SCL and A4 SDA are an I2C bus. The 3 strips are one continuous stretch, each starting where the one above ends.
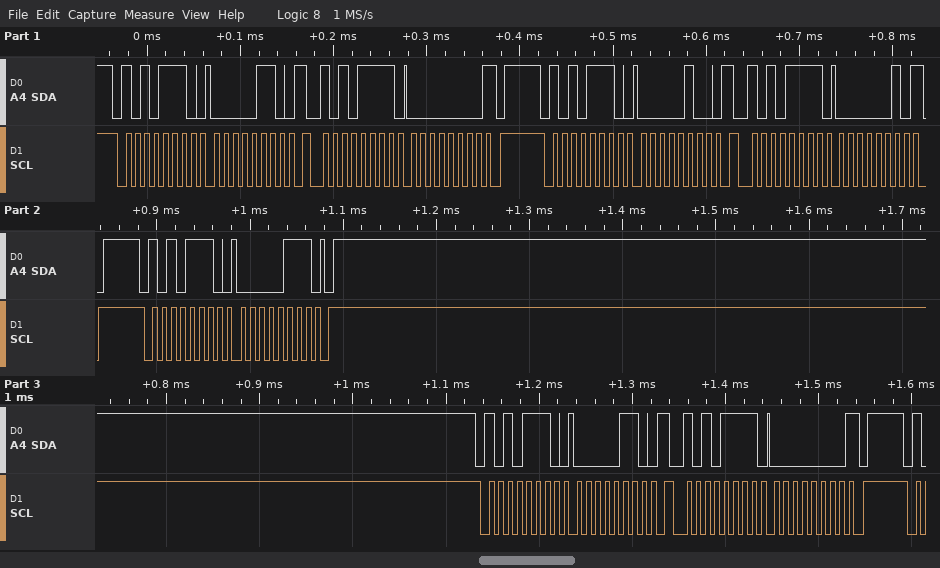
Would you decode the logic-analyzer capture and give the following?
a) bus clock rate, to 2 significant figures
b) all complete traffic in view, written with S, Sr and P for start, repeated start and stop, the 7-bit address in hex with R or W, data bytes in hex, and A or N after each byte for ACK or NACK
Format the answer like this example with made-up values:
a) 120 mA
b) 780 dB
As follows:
a) 100 kHz
b) S 57W A 06 A Sr 57R A 00 N P S 57W A 04 A Sr 57R A 02 N P S 57W A 07 A P S 57W A 06 A Sr 57R A 00 N P
